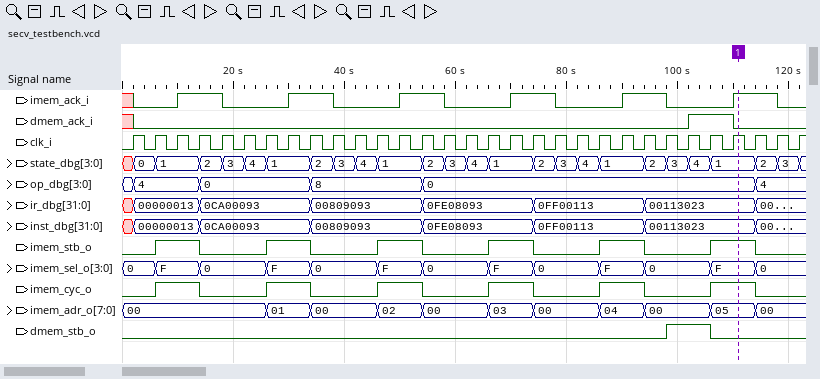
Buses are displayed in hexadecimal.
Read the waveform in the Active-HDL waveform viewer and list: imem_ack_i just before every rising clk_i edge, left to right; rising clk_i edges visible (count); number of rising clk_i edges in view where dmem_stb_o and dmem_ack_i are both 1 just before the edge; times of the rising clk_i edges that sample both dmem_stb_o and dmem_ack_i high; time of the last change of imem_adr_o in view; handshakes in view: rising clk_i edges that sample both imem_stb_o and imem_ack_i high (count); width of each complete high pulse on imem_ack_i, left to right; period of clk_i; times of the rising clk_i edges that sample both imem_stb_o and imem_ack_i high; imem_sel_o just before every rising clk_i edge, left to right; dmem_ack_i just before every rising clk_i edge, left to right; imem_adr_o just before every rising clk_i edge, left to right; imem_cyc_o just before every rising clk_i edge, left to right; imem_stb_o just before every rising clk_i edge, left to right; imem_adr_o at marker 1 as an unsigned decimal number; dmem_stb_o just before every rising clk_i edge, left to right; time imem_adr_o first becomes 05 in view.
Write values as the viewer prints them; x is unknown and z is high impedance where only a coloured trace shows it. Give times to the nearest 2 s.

x 0 0 1 1 0 0 0 1 1 0 0 0 1 1 0 0 0 1 1 0 0 0 1 1 0 0 0 1 1 0
31
1
106 s
114 s
6
8 s, 8 s, 8 s, 8 s, 8 s, 8 s
4 s
14 s, 34 s, 54 s, 74 s, 94 s, 114 s
0, 0, F, F, 0, 0, 0, F, F, 0, 0, 0, F, F, 0, 0, 0, F, F, 0, 0, 0, F, F, 0, 0, 0, F, F, 0, 0
x 0 0 0 0 0 0 0 0 0 0 0 0 0 0 0 0 0 0 0 0 0 0 0 0 0 1 1 0 0 0
00, 00, 00, 00, 00, 00, 00, 01, 01, 00, 00, 00, 02, 02, 00, 00, 00, 03, 03, 00, 00, 00, 04, 04, 00, 00, 00, 05, 05, 00, 00
0 0 1 1 0 0 0 1 1 0 0 0 1 1 0 0 0 1 1 0 0 0 1 1 0 0 0 1 1 0 0
0 0 1 1 0 0 0 1 1 0 0 0 1 1 0 0 0 1 1 0 0 0 1 1 0 0 0 1 1 0 0
5
0 0 0 0 0 0 0 0 0 0 0 0 0 0 0 0 0 0 0 0 0 0 0 0 0 1 1 0 0 0 0
106 s
